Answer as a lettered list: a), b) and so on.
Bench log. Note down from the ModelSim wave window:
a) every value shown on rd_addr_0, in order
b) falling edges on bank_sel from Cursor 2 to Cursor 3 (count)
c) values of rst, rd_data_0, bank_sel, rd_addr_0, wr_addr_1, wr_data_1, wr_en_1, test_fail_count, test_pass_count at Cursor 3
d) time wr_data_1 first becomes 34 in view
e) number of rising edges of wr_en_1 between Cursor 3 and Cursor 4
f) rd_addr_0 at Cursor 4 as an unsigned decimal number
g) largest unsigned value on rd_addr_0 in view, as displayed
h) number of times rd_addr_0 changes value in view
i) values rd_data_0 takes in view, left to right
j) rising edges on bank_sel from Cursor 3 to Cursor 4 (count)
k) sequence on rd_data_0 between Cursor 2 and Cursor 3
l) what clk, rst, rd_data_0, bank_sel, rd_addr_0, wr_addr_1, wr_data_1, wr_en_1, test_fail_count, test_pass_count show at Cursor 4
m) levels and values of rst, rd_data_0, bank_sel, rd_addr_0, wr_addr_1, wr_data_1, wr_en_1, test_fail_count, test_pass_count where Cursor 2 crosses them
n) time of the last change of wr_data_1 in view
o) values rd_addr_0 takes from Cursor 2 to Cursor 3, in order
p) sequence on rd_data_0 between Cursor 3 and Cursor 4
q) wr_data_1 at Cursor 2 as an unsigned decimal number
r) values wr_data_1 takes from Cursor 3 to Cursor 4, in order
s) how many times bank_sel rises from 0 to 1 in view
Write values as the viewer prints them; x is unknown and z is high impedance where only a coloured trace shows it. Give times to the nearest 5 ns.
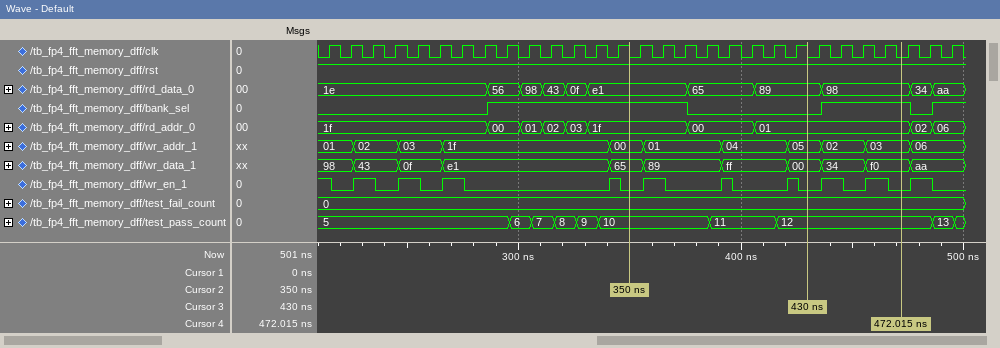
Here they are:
a) 1f, 00, 01, 02, 03, 1f, 00, 01, 02, 06
b) 1
c) rst=1, rd_data_0=89, bank_sel=0, rd_addr_0=01, wr_addr_1=05, wr_data_1=00, wr_en_1=0, test_fail_count=0, test_pass_count=12
d) 435 ns
e) 2
f) 1
g) 1f
h) 9
i) 1e, 56, 98, 43, 0f, e1, 65, 89, 98, 34, aa
j) 1
k) e1, 65, 89
l) clk=0, rst=1, rd_data_0=98, bank_sel=1, rd_addr_0=01, wr_addr_1=03, wr_data_1=f0, wr_en_1=0, test_fail_count=0, test_pass_count=12
m) rst=1, rd_data_0=e1, bank_sel=1, rd_addr_0=1f, wr_addr_1=00, wr_data_1=65, wr_en_1=0, test_fail_count=0, test_pass_count=10
n) 475 ns
o) 1f, 00, 01
p) 89, 98
q) 101
r) 00, 34, f0
s) 3
